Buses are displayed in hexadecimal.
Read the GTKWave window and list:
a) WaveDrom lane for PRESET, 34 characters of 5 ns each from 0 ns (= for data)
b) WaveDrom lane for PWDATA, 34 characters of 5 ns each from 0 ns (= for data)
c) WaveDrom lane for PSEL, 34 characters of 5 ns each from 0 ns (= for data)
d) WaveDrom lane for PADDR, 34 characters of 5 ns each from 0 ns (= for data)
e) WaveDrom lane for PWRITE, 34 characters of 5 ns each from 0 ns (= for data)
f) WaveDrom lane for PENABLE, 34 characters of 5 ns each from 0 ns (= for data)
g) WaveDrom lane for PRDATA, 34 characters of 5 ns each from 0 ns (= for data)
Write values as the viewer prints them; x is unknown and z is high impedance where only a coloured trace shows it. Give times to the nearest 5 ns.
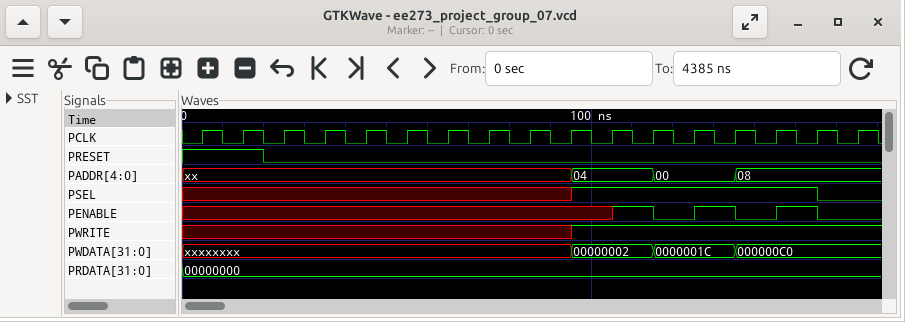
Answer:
{name: 'PRESET', wave: '1...0.............................'}
{name: 'PWDATA', wave: 'x..................=...=...=......', data: '00000002 0000001C 000000C0'}
{name: 'PSEL', wave: 'x..................1...........0..'}
{name: 'PADDR', wave: 'x..................=...=...=......', data: '04 00 08'}
{name: 'PWRITE', wave: 'x..................1..............'}
{name: 'PENABLE', wave: 'x....................1.0.1.0.1.0..'}
{name: 'PRDATA', wave: '=.................................', data: '00000000'}
